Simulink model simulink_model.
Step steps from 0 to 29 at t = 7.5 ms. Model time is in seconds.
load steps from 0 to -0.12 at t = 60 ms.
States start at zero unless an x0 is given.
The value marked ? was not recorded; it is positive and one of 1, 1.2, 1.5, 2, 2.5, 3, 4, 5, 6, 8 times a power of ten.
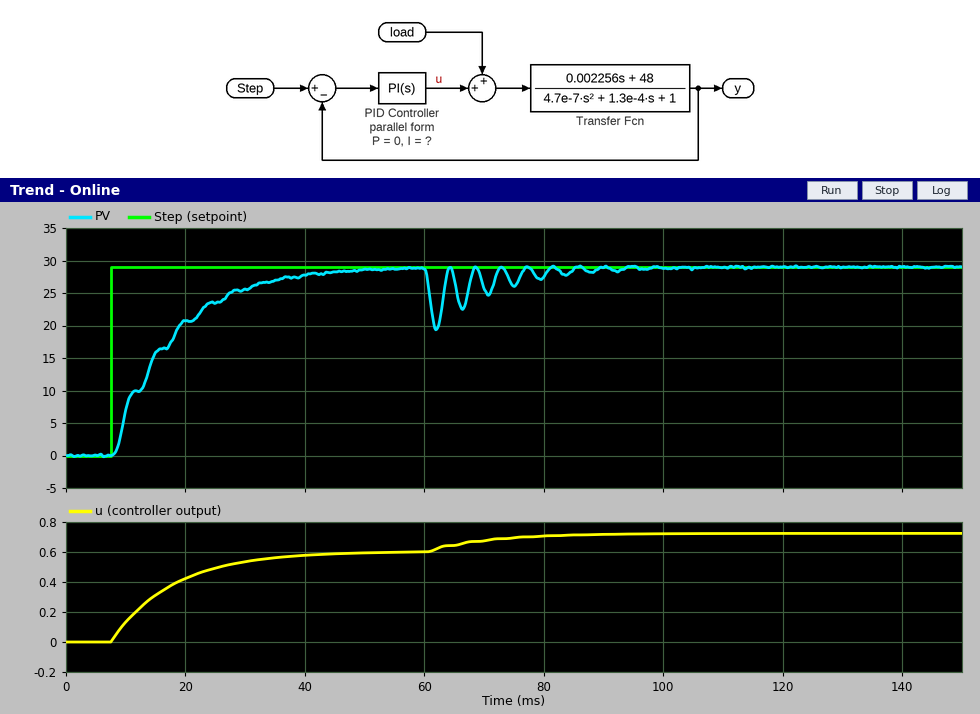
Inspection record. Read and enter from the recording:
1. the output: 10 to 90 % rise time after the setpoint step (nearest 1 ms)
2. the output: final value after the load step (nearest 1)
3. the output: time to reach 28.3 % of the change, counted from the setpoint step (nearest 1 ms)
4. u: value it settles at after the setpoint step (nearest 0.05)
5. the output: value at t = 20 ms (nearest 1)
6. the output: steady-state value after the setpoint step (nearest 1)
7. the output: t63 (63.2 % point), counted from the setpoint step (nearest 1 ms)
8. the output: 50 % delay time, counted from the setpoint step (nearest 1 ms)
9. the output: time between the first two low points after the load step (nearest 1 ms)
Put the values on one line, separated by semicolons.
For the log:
22 ms; 29; 3 ms; 0.60; 21; 29; 11 ms; 7 ms; 4 ms
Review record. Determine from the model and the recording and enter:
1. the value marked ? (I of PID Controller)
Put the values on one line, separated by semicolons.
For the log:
2
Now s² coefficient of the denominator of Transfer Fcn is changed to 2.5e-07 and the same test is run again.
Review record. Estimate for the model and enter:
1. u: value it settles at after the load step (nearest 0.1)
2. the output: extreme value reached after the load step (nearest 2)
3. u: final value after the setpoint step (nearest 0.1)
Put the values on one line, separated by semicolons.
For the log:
0.7; 20; 0.6
